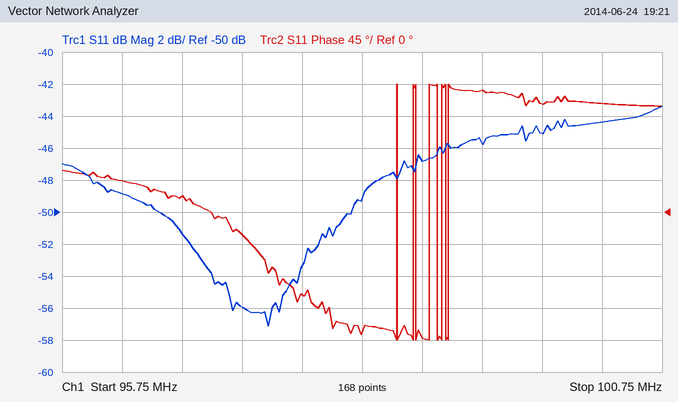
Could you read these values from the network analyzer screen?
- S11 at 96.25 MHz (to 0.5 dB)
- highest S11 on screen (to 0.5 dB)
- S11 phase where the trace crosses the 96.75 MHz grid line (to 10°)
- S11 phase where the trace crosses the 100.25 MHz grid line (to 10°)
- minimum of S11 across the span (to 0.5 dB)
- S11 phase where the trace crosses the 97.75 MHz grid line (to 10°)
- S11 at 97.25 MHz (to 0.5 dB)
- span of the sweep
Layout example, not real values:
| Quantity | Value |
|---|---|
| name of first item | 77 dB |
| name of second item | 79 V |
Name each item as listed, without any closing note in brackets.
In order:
| Quantity | Value |
|---|---|
| S11 at 96.25 MHz | -49.0 dB |
| highest S11 on screen | -43.5 dB |
| S11 phase where the trace crosses the 96.75 MHz grid line | 20° |
| S11 phase where the trace crosses the 100.25 MHz grid line | 150° |
| minimum of S11 across the span | -57.0 dB |
| S11 phase where the trace crosses the 97.75 MHz grid line | -120° |
| S11 at 97.25 MHz | -56.0 dB |
| span of the sweep | 5 MHz |
